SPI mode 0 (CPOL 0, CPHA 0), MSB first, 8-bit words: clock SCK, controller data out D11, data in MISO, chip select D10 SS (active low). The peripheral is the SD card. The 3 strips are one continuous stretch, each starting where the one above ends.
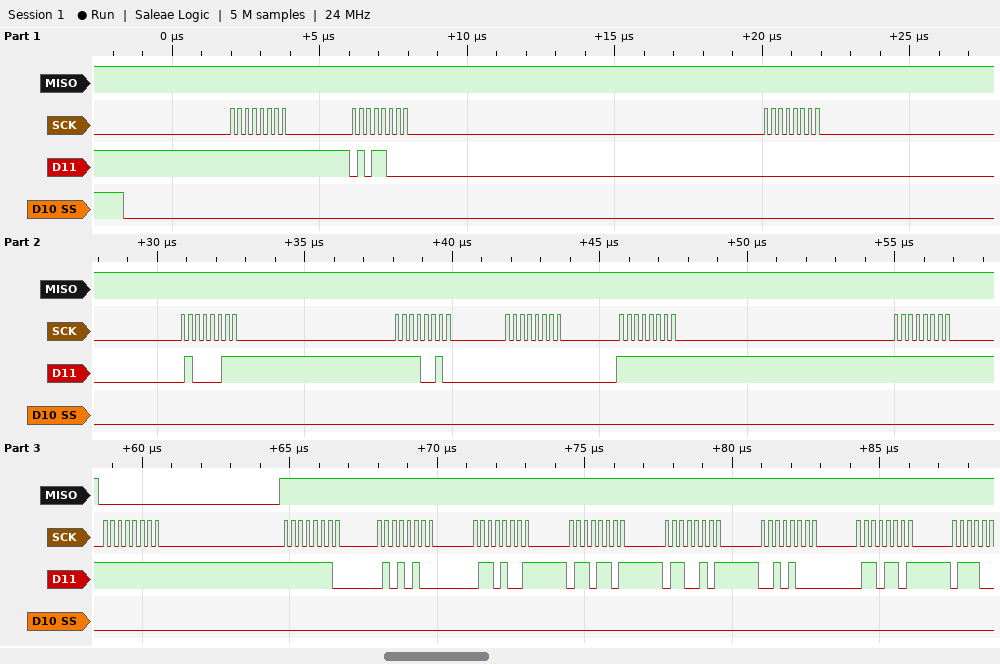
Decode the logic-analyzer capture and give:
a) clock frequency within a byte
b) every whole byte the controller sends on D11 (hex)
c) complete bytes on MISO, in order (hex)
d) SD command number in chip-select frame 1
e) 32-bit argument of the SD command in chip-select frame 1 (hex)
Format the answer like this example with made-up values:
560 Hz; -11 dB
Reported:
4 MHz; FF 58 00 43 F2 00 FF FF FF FE 54 69 6D 65 28 6D; FF FF FF FF FF FF FF FF 00 FF FF FF FF FF FF FF; CMD24; 0x0043F200
